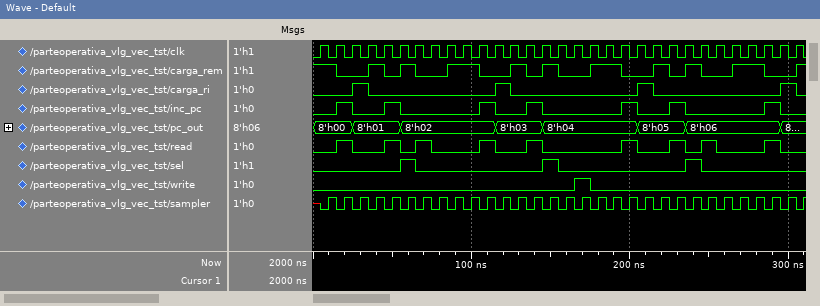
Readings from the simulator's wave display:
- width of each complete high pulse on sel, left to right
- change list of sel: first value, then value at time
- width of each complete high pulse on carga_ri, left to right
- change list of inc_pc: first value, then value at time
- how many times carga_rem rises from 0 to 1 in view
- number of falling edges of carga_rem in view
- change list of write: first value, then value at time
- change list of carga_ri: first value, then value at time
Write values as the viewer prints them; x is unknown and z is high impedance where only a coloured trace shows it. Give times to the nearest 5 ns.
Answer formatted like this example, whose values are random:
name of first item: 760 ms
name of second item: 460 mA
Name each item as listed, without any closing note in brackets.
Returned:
width of each complete high pulse on sel, left to right: 10 ns, 10 ns, 10 ns
change list of sel: first value, then value at time: 0, 1 at 55 ns, 0 at 65 ns, 1 at 145 ns, 0 at 155 ns, 1 at 235 ns, 0 at 245 ns
width of each complete high pulse on carga_ri, left to right: 10 ns, 10 ns, 10 ns, 10 ns
change list of inc_pc: first value, then value at time: 0, 1 at 15 ns, 0 at 25 ns, 1 at 45 ns, 0 at 55 ns, 1 at 105 ns, 0 at 115 ns, 1 at 135 ns, 0 at 145 ns, 1 at 195 ns, 0 at 205 ns, 1 at 225 ns, 0 at 235 ns, 1 at 285 ns, 0 at 295 ns
how many times carga_rem rises from 0 to 1 in view: 10
number of falling edges of carga_rem in view: 10
change list of write: first value, then value at time: 0, 1 at 165 ns, 0 at 175 ns
change list of carga_ri: first value, then value at time: 0, 1 at 25 ns, 0 at 35 ns, 1 at 115 ns, 0 at 125 ns, 1 at 205 ns, 0 at 215 ns, 1 at 295 ns, 0 at 305 ns
